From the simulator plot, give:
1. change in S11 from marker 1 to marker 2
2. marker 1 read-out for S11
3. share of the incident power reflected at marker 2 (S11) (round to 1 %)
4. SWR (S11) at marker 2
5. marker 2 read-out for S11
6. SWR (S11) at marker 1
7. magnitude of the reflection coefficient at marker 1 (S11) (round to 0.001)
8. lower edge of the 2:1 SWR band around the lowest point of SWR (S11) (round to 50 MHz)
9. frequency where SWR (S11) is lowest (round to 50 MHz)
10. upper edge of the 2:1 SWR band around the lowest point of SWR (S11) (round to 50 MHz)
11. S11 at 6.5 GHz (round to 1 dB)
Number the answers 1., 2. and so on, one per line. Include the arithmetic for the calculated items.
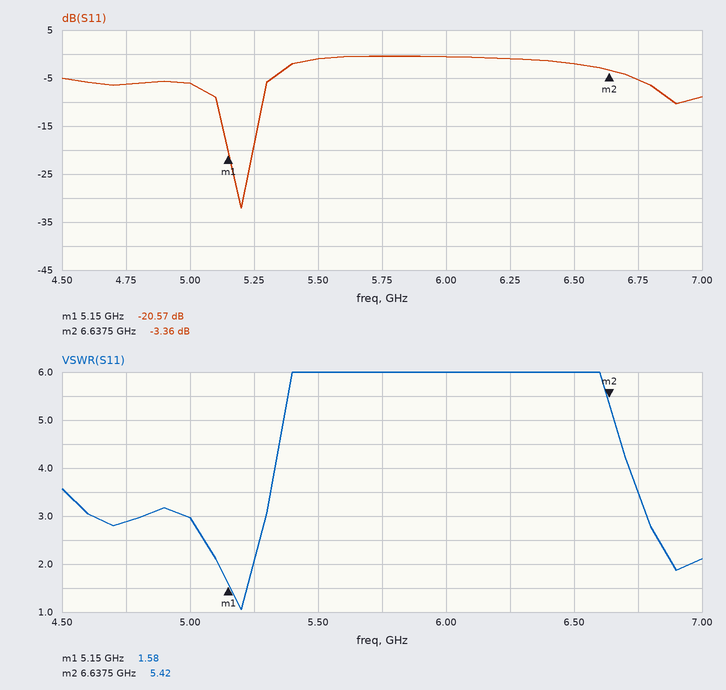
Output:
1. -3.36 − (-20.57) = 17.21 dB
2. -20.57 dB
3. 10^(-3.36/10) ≈ 46 %
4. 5.42
5. -3.36 dB
6. 1.58
7. 10^(-20.57/20) ≈ 0.094
8. 5.10 GHz
9. 5.20 GHz
10. 5.25 GHz
11. -2 dB
